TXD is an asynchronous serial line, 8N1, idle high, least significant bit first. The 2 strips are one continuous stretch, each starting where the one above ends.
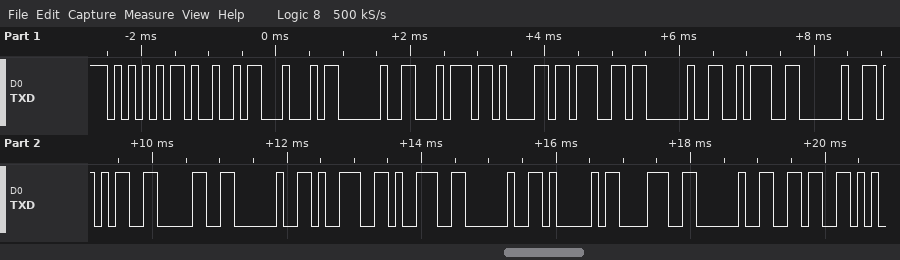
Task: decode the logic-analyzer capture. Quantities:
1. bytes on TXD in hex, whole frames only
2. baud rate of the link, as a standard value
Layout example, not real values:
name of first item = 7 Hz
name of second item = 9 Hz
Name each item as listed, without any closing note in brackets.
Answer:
bytes on TXD in hex, whole frames only = 0x55 0x49 0x44 0x20 0x74 0x61 0x67 0x20 0x3A 0x20 0x35 0x30 0x20 0x39 0x39 0x20 0x41 0x38 0x20 0x36
baud rate of the link, as a standard value = 9600 baud
